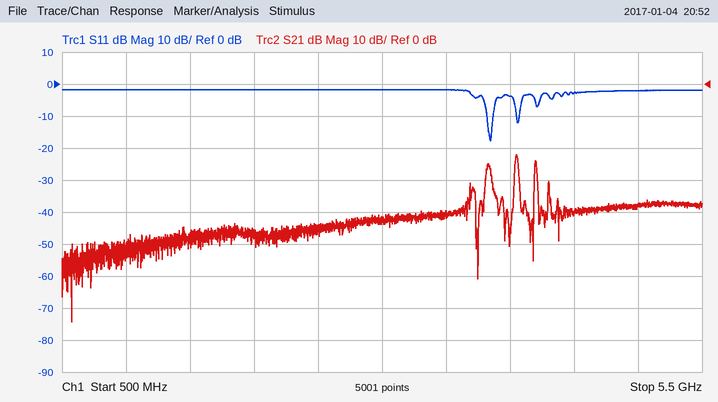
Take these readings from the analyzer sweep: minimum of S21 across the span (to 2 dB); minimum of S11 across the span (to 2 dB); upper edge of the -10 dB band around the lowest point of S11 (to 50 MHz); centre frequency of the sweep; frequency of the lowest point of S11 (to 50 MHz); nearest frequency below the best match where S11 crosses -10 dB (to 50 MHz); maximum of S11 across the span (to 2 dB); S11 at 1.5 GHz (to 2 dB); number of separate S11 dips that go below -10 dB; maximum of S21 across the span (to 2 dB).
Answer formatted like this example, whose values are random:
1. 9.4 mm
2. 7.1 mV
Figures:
1. -74 dB
2. -18 dB
3. 3.85 GHz
4. 3 GHz
5. 3.85 GHz
6. 3.80 GHz
7. -2 dB
8. -2 dB
9. 2
10. -22 dB
